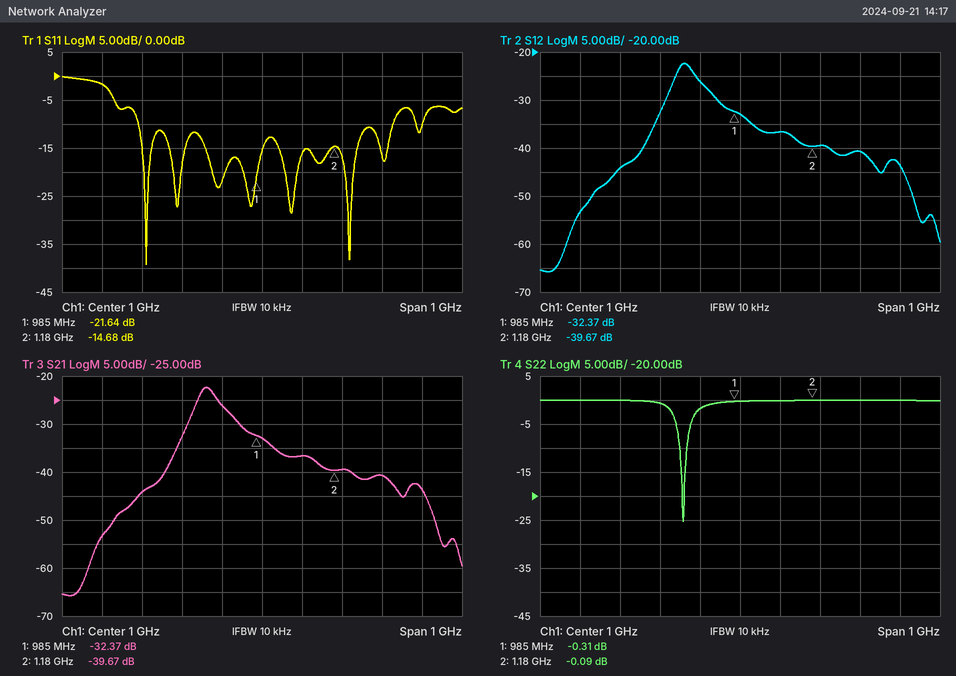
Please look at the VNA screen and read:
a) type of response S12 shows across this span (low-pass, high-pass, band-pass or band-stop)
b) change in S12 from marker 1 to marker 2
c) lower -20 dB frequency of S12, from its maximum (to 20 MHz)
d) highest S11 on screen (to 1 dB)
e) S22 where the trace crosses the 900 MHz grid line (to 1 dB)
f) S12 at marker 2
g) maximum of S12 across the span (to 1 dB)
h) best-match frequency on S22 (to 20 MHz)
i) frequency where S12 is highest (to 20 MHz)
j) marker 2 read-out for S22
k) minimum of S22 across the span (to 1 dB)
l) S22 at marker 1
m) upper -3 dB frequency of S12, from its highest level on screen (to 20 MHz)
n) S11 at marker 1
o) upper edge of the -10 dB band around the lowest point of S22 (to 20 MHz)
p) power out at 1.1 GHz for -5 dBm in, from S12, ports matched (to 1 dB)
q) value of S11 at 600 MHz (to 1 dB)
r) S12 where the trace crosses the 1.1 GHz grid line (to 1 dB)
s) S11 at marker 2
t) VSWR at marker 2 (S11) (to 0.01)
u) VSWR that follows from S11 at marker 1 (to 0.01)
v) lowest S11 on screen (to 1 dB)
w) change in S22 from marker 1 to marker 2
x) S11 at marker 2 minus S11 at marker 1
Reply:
band-pass
-7.30 dB
740 MHz
0 dB
-2 dB
-39.67 dB
-22 dB
860 MHz
860 MHz
-0.09 dB
-25 dB
-0.31 dB
900 MHz
-21.64 dB
860 MHz
-42 dBm
-2 dB
-37 dB
-14.68 dB
1.45
1.18
-39 dB
0.22 dB
6.96 dB
